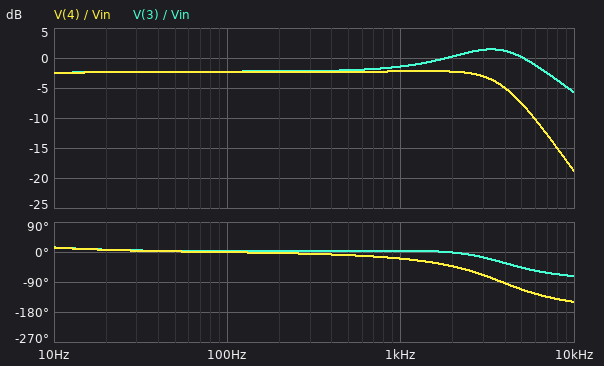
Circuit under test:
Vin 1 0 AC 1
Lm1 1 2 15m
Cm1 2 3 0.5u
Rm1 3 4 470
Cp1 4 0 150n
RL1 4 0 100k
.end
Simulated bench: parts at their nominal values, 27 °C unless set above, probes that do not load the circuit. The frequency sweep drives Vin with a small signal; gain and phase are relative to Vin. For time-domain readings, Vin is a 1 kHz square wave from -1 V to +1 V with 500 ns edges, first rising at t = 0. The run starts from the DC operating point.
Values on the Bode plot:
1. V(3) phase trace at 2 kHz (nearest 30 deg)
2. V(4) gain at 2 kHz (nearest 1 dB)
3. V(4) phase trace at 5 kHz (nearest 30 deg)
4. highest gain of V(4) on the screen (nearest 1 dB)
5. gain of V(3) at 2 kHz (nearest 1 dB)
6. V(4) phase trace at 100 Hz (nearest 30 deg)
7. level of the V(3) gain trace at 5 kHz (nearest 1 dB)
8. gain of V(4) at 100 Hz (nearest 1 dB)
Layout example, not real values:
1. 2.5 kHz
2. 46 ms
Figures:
1. 0 deg
2. -2 dB
3. -120 deg
4. -2 dB
5. 0 dB
6. 0 deg
7. 0 dB
8. -2 dB
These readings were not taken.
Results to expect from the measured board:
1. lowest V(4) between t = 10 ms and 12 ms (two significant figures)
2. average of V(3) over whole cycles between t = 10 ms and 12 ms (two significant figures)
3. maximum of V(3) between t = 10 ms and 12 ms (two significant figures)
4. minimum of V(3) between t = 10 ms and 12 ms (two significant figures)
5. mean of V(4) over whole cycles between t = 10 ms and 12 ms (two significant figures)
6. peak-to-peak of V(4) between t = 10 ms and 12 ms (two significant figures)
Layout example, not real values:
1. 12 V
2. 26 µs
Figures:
1. -230 mV
2. 650 mV
3. 2.0 V
4. -680 mV
5. 650 mV
6. 1.8 V
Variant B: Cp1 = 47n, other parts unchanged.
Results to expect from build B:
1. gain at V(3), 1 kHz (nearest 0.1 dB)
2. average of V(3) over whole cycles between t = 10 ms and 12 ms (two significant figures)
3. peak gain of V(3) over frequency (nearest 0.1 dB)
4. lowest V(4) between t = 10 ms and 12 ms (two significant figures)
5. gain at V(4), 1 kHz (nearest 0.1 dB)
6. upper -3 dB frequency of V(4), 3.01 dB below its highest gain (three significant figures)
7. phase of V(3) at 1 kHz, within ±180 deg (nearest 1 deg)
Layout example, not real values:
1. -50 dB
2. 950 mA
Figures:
1. -0.5 dB
2. 750 mV
3. 3.9 dB
4. -640 mV
5. -0.7 dB
6. 7.47 kHz
7. 1 deg
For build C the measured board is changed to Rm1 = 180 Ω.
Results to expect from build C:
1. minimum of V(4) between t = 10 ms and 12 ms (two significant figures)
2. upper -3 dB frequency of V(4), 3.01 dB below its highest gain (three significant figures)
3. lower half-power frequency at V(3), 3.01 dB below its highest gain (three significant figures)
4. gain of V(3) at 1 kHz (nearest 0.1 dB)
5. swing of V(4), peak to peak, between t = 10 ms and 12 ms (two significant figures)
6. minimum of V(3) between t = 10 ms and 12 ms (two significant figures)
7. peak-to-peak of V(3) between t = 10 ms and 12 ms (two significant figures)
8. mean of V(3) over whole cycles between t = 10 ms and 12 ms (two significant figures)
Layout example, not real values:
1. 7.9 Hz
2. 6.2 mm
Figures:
1. -800 mV
2. 4.46 kHz
3. 2.59 kHz
4. -1.6 dB
5. 2.9 V
6. -960 mV
7. 3.2 V
8. 650 mV
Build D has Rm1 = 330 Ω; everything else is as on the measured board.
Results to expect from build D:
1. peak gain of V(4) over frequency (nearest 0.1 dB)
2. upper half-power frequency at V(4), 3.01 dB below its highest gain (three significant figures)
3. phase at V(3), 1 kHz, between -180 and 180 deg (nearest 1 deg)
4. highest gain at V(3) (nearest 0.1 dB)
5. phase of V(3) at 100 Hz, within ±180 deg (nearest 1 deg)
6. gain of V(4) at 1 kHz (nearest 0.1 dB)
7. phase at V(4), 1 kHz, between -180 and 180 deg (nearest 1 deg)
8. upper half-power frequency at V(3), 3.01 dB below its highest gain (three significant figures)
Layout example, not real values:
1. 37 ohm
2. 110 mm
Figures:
1. -0.5 dB
2. 4.52 kHz
3. 3 deg
4. 2.5 dB
5. 2 deg
6. -2.0 dB
7. -14 deg
8. 5.32 kHz
